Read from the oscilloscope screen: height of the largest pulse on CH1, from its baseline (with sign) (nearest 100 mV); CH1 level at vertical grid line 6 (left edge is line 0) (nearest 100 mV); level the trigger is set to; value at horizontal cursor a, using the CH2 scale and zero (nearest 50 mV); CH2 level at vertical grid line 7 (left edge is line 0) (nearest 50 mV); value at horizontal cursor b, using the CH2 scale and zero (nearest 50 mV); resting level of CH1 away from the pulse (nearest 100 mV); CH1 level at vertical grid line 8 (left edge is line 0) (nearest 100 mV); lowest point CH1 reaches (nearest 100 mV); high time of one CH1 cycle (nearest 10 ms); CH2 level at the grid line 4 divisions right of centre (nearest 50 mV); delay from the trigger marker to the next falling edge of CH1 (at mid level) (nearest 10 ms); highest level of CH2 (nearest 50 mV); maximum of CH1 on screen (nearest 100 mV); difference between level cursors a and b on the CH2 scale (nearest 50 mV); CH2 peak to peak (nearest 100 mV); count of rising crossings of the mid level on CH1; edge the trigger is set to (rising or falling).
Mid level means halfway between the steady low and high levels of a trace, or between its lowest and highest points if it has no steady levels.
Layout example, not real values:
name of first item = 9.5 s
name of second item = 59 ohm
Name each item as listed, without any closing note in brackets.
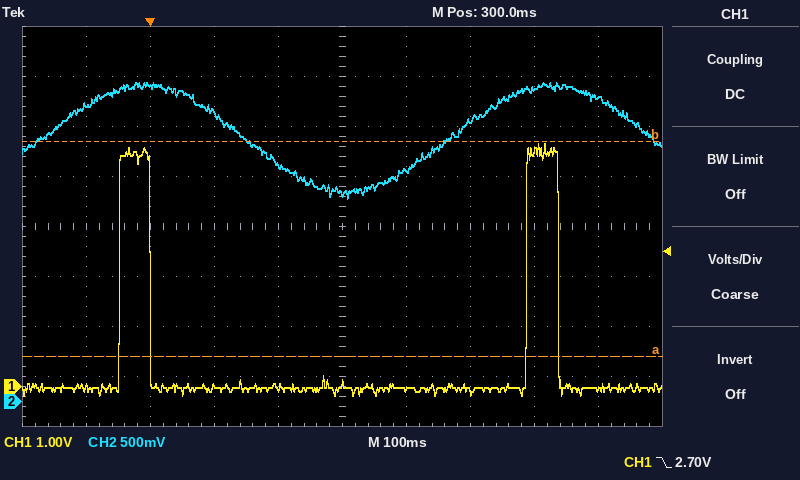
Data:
height of the largest pulse on CH1, from its baseline (with sign) = +4.9 V
CH1 level at vertical grid line 6 (left edge is line 0) = -100 mV
level the trigger is set to = 2.70 V
value at horizontal cursor a, using the CH2 scale and zero = 450 mV
CH2 level at vertical grid line 7 (left edge is line 0) = 2.80 V
value at horizontal cursor b, using the CH2 scale and zero = 2.60 V
resting level of CH1 away from the pulse = 0.0 V
CH1 level at vertical grid line 8 (left edge is line 0) = 4.7 V
lowest point CH1 reaches = -200 mV
high time of one CH1 cycle = 50 ms
CH2 level at the grid line 4 divisions right of centre = 3.05 V
delay from the trigger marker to the next falling edge of CH1 (at mid level) = 640 ms
highest level of CH2 = 3.20 V
maximum of CH1 on screen = 4.9 V
difference between level cursors a and b on the CH2 scale = 2.15 V
CH2 peak to peak = 1.20 V
count of rising crossings of the mid level on CH1 = 2
edge the trigger is set to = falling
